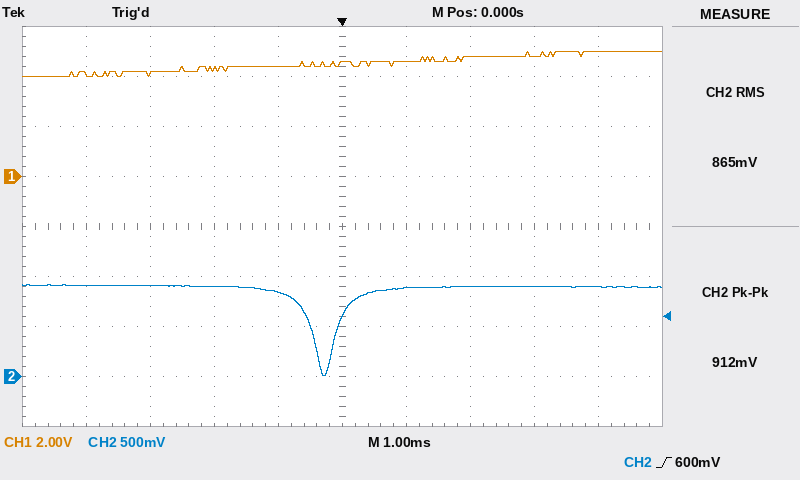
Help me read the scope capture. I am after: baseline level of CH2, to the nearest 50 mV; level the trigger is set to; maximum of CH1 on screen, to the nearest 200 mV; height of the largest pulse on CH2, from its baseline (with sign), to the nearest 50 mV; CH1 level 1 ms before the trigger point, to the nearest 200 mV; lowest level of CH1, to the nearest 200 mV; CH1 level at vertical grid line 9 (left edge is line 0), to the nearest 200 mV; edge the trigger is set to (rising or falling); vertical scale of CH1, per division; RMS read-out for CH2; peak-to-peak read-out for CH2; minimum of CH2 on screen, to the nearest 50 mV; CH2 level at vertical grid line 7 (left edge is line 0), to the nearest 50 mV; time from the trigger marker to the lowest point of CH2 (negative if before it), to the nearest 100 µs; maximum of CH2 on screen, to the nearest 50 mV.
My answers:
900 mV
600 mV
5.0 V
-900 mV
4.4 V
4.0 V
5.0 V
rising
2 V
865 mV
912 mV
0 mV
900 mV
-300 µs
900 mV
